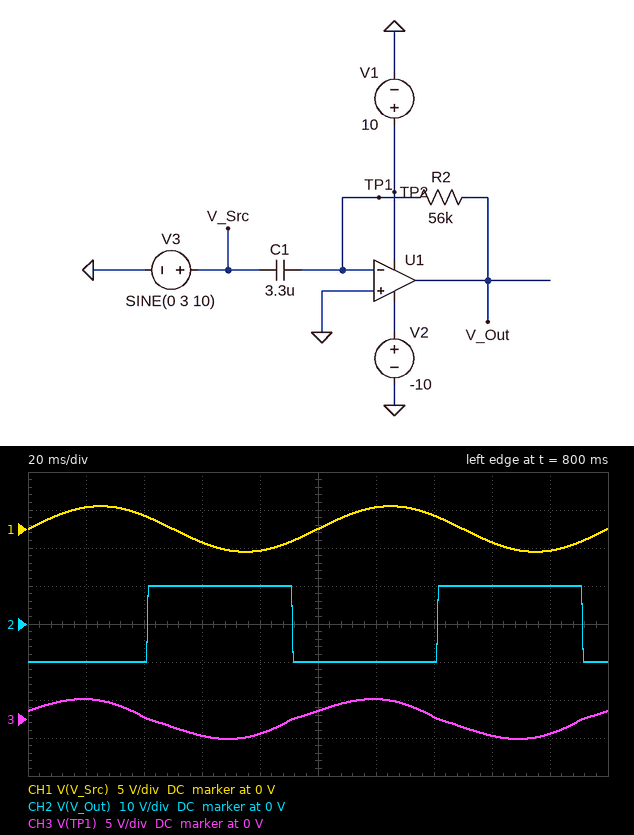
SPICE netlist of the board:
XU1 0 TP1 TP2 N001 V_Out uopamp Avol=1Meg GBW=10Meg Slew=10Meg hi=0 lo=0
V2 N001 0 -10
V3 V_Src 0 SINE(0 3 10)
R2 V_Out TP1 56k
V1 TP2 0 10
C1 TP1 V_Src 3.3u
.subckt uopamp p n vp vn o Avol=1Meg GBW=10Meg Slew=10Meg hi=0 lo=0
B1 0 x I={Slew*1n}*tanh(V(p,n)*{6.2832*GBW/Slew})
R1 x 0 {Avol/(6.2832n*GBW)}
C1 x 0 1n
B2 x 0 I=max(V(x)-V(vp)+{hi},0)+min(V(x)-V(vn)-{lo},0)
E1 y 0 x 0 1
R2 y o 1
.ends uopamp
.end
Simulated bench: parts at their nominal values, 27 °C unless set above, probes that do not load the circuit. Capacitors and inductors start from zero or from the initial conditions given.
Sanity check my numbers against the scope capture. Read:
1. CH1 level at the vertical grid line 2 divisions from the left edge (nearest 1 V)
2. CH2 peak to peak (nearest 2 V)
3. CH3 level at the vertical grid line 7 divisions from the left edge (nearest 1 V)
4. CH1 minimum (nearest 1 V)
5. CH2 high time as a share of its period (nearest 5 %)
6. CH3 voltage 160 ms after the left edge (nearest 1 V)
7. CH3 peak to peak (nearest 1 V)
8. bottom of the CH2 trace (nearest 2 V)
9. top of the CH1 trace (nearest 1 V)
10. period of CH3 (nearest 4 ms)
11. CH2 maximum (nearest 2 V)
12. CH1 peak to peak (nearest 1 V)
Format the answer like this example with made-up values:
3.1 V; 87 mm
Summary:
2 V; 20 V; 0 V; -3 V; 50 %; -2 V; 5 V; -10 V; 3 V; 100 ms; 10 V; 6 V
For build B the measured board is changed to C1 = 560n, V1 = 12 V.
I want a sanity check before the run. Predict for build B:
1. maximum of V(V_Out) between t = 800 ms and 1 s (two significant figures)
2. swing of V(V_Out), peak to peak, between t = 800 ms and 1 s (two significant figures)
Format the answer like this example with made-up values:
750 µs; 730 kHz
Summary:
5.9 V; 12 V
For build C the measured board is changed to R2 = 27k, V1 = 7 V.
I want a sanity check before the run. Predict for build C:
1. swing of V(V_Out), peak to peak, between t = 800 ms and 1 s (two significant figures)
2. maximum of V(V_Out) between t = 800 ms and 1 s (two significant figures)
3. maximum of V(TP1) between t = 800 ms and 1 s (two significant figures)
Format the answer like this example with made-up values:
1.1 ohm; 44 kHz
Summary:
17 V; 7.0 V; 1.3 V
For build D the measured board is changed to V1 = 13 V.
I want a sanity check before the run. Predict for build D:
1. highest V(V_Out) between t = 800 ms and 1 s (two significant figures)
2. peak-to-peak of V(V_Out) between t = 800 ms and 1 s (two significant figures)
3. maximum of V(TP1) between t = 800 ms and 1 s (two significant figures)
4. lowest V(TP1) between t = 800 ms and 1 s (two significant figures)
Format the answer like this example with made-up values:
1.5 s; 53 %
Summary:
13 V; 23 V; 2.9 V; -2.1 V
